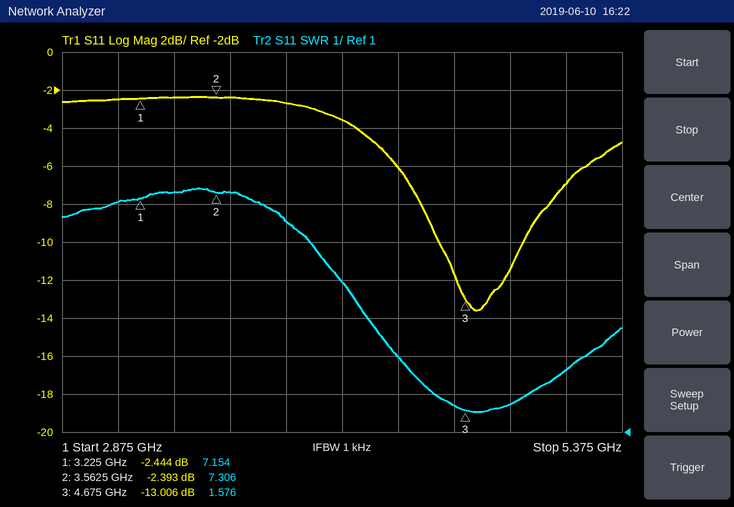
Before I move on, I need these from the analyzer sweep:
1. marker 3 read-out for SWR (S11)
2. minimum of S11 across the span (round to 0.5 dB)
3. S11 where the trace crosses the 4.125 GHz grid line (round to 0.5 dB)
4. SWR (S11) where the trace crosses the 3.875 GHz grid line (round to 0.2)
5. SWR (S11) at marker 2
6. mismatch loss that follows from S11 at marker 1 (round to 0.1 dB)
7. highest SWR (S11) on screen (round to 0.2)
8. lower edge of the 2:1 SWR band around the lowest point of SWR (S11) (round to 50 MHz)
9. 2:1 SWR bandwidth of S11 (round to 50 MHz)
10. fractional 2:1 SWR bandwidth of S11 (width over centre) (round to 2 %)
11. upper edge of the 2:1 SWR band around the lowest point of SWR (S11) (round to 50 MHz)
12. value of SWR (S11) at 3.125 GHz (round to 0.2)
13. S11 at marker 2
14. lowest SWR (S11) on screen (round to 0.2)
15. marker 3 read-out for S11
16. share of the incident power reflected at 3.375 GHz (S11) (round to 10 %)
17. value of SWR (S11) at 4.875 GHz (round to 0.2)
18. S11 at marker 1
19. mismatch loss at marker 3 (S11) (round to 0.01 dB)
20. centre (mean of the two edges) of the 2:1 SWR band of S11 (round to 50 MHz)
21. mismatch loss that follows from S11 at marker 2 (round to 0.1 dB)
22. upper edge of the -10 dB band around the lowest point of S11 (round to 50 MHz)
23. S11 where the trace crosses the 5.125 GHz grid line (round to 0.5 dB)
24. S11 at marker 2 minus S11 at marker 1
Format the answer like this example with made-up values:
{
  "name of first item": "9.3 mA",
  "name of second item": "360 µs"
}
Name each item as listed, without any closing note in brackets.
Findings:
{
  "marker 3 read-out for SWR": "1.576",
  "minimum of S11 across the span": "-13.5 dB",
  "S11 where the trace crosses the 4.125 GHz grid line": "-3.5 dB",
  "SWR (S11) where the trace crosses the 3.875 GHz grid line": "6.6",
  "SWR (S11) at marker 2": "7.306",
  "mismatch loss that follows from S11 at marker 1": "3.7 dB",
  "highest SWR (S11) on screen": "7.4",
  "lower edge of the 2:1 SWR band around the lowest point of SWR (S11)": "4.55 GHz",
  "2:1 SWR bandwidth of S11": "400 MHz",
  "fractional 2:1 SWR bandwidth of S11 (width over centre)": "8 %",
  "upper edge of the 2:1 SWR band around the lowest point of SWR (S11)": "4.95 GHz",
  "value of SWR (S11) at 3.125 GHz": "7.0",
  "S11 at marker 2": "-2.393 dB",
  "lowest SWR (S11) on screen": "1.6",
  "marker 3 read-out for S11": "-13.006 dB",
  "share of the incident power reflected at 3.375 GHz (S11)": "60 %",
  "value of SWR (S11) at 4.875 GHz": "1.8",
  "S11 at marker 1": "-2.444 dB",
  "mismatch loss at marker 3 (S11)": "0.22 dB",
  "centre (mean of the two edges) of the 2:1 SWR band of S11": "4.75 GHz",
  "mismatch loss that follows from S11 at marker 2": "3.7 dB",
  "upper edge of the -10 dB band around the lowest point of S11": "4.95 GHz",
  "S11 where the trace crosses the 5.125 GHz grid line": "-7.0 dB",
  "S11 at marker 2 minus S11 at marker 1": "0.051 dB"
}
